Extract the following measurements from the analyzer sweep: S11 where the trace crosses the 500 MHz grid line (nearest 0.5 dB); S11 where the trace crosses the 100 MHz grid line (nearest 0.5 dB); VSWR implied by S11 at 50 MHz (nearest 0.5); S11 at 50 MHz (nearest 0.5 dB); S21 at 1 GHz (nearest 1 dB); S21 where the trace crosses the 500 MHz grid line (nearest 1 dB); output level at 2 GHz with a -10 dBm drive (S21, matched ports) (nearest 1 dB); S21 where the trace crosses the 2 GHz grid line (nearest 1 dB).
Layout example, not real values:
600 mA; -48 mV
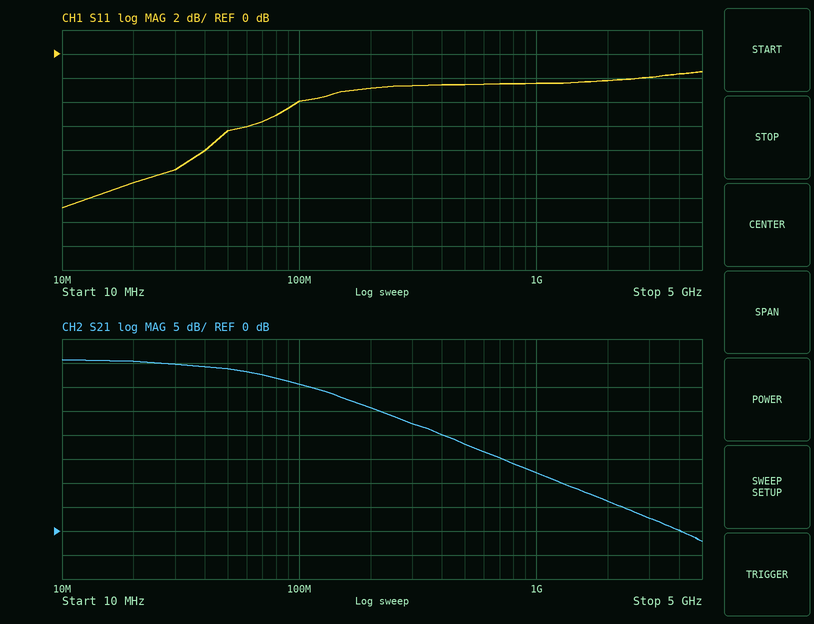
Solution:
-2.5 dB; -4.0 dB; 3.0; -6.5 dB; 12 dB; 18 dB; -4 dBm; 6 dB
